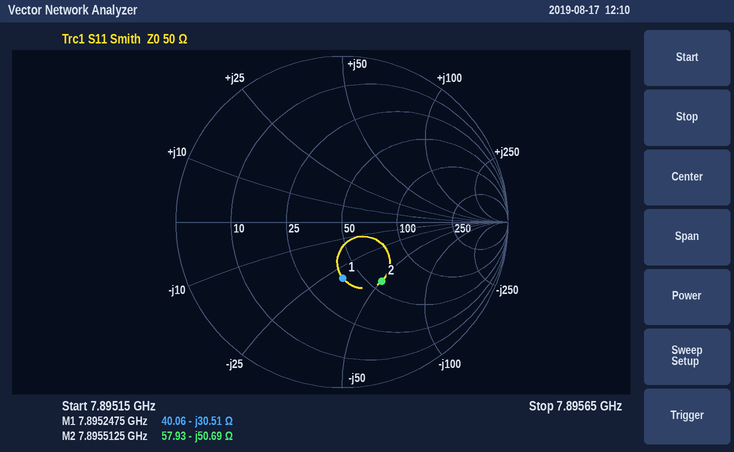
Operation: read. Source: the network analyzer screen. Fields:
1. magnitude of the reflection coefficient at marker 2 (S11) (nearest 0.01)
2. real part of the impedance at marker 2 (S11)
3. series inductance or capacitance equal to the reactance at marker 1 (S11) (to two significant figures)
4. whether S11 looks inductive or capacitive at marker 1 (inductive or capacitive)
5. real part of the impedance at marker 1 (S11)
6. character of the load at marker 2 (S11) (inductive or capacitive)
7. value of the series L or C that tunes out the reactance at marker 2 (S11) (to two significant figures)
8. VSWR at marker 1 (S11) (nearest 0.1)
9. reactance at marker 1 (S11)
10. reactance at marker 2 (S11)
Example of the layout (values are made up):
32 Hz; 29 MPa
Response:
0.43; 57.93 Ω; 660 fF; capacitive; 40.06 Ω; capacitive; 1.0 nH; 2.0; -30.51 Ω; -50.69 Ω
